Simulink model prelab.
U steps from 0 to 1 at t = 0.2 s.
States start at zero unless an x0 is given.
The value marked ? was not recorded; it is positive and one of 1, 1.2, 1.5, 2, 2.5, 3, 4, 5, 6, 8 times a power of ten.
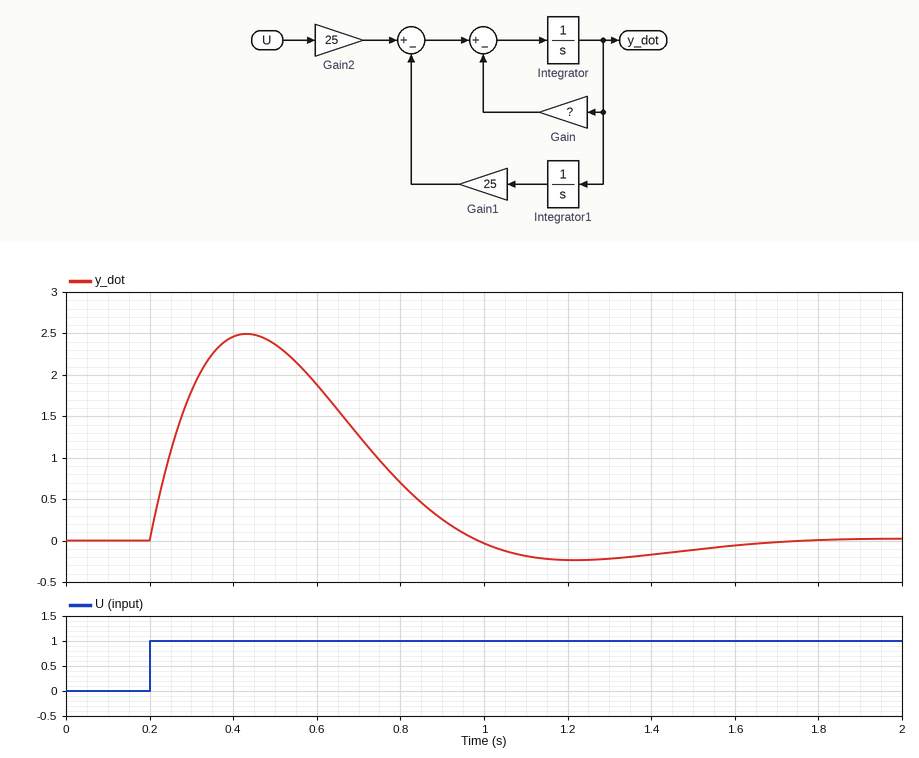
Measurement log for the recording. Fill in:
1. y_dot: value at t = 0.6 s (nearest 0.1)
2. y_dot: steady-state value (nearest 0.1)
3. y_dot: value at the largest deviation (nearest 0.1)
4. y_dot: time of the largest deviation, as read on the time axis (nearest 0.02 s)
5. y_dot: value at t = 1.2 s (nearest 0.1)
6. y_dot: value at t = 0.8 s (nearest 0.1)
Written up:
1.9
0.0
2.5
0.44 s
-0.2
0.7
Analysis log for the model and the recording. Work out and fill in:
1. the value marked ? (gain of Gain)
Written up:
6
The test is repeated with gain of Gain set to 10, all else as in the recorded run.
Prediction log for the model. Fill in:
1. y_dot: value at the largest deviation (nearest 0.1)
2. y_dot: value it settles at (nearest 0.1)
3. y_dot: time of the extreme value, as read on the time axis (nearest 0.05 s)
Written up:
1.8
0.0
0.40 s
